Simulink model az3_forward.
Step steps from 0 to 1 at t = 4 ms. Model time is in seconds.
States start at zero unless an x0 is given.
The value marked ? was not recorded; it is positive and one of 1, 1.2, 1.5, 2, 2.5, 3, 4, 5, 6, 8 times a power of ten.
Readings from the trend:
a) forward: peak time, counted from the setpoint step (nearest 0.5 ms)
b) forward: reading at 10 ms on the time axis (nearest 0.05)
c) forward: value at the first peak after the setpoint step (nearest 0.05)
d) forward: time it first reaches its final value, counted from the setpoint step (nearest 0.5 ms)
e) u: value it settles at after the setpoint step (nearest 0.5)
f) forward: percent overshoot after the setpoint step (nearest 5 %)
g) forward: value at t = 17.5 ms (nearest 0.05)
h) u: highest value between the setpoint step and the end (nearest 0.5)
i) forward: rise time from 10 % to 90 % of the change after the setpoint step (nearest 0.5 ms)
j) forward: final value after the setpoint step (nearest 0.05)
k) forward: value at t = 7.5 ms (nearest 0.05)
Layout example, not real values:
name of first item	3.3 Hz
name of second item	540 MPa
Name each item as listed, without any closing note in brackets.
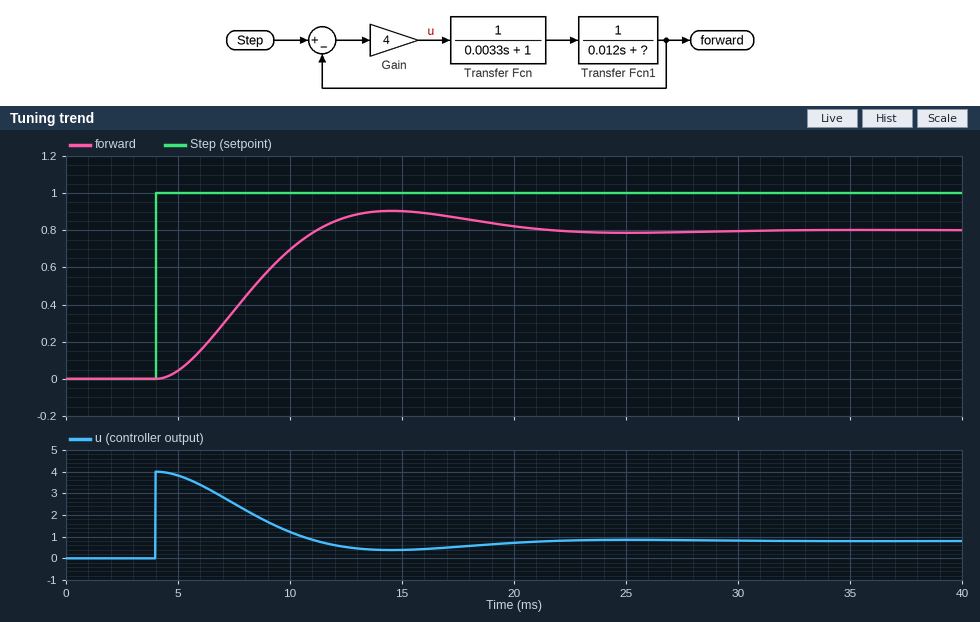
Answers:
forward: peak time, counted from the setpoint step	10.5 ms
forward: reading at 10 ms on the time axis	0.70
forward: value at the first peak after the setpoint step	0.90
forward: time it first reaches its final value, counted from the setpoint step	7.0 ms
u: value it settles at after the setpoint step	1.0
forward: percent overshoot after the setpoint step	15 %
forward: value at t = 17.5 ms	0.85
u: highest value between the setpoint step and the end	4.0
forward: rise time from 10 % to 90 % of the change after the setpoint step	5.0 ms
forward: final value after the setpoint step	0.80
forward: value at t = 7.5 ms	0.35
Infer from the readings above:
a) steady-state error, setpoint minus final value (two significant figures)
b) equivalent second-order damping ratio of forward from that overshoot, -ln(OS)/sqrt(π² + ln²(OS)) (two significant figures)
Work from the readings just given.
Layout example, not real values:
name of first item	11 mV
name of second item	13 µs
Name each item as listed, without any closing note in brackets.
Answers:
steady-state error, setpoint minus final value	0.20
equivalent second-order damping ratio of forward from that overshoot, -ln(OS)/sqrt(π² + ln²(OS))	0.52
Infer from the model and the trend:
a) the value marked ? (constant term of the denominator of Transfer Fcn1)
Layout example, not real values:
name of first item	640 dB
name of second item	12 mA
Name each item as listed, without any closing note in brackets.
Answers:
the value marked ?	1
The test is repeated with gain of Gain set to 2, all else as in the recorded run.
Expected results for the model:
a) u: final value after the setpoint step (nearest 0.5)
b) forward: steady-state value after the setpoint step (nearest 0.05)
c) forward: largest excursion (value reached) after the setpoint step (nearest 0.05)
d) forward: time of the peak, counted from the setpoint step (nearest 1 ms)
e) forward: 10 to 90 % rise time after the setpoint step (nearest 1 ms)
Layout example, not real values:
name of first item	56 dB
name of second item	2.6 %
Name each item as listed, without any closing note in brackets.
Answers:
u: final value after the setpoint step	0.5
forward: steady-state value after the setpoint step	0.65
forward: largest excursion (value reached) after the setpoint step	0.70
forward: time of the peak, counted from the setpoint step	16 ms
forward: 10 to 90 % rise time after the setpoint step	8 ms
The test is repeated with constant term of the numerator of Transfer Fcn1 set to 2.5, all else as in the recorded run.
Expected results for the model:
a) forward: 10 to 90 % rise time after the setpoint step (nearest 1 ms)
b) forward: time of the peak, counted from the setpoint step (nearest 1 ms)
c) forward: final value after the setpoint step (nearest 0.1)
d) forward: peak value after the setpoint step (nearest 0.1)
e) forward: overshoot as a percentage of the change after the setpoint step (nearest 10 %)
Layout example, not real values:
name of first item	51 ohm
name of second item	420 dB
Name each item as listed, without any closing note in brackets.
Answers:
forward: 10 to 90 % rise time after the setpoint step	3 ms
forward: time of the peak, counted from the setpoint step	6 ms
forward: final value after the setpoint step	0.9
forward: peak value after the setpoint step	1.2
forward: overshoot as a percentage of the change after the setpoint step	30 %
